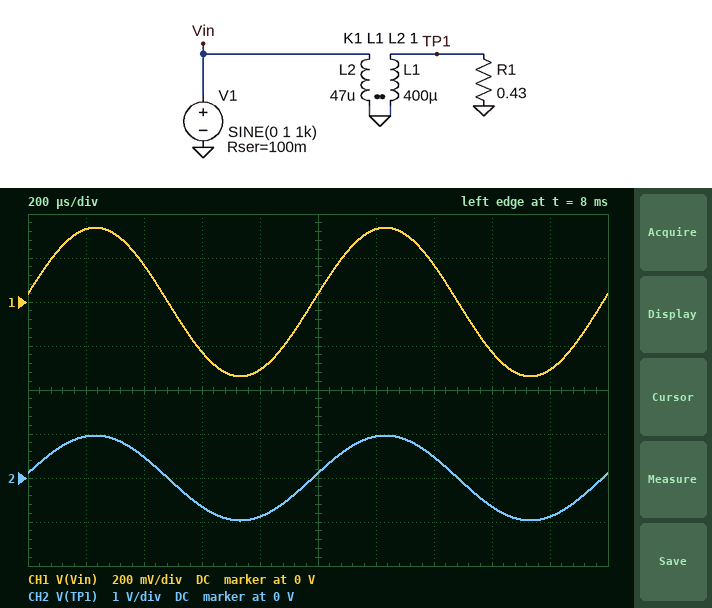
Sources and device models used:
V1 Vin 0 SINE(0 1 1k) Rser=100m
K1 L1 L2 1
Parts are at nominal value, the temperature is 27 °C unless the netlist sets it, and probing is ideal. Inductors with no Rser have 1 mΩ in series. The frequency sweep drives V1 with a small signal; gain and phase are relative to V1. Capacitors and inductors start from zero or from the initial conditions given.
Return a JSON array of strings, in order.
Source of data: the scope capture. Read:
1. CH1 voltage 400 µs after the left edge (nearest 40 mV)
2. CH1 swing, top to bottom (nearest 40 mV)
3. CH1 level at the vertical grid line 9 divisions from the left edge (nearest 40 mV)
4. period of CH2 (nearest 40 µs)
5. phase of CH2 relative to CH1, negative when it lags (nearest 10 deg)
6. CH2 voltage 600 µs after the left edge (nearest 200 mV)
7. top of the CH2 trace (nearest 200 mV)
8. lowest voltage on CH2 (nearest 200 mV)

["160 mV", "680 mV", "-320 mV", "1.00 ms", "0 deg", "-600 mV", "1.0 V", "-1.0 V"]
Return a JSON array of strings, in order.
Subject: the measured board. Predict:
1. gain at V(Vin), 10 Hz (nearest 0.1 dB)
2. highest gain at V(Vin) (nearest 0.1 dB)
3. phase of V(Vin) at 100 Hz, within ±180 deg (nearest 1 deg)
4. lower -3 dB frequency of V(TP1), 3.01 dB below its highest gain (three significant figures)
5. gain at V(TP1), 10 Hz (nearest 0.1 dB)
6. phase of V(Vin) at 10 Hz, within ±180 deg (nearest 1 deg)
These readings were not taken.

["-30.1 dB", "-9.4 dB", "47 deg", "114 Hz", "-21.4 dB", "67 deg"]
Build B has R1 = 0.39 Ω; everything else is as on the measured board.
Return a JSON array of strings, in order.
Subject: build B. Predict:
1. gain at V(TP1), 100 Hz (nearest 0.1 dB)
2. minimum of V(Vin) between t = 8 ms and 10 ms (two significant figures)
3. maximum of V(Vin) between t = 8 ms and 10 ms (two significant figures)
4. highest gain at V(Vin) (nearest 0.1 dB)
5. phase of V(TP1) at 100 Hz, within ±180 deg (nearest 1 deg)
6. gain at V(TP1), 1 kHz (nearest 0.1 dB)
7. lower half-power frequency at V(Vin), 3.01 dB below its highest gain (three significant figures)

["-4.1 dB", "-320 mV", "320 mV", "-9.9 dB", "47 deg", "-0.9 dB", "107 Hz"]
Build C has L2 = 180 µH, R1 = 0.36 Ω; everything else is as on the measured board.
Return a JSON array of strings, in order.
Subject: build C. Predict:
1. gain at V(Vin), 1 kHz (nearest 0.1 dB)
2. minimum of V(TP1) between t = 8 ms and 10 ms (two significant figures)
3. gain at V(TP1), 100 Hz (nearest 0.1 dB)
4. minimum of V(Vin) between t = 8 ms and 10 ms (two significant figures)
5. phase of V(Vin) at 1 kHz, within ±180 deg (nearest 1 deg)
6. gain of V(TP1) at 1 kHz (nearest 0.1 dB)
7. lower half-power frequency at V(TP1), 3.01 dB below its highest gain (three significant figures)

["-4.2 dB", "-920 mV", "-1.9 dB", "-620 mV", "3 deg", "-0.8 dB", "55.1 Hz"]
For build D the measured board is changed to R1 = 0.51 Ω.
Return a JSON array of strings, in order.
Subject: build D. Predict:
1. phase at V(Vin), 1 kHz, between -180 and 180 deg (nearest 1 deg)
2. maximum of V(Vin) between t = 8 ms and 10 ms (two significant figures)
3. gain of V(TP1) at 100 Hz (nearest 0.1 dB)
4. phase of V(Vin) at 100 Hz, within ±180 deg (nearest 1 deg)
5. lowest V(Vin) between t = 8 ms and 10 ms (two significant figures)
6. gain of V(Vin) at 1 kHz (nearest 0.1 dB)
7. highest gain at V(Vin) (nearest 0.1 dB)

["7 deg", "380 mV", "-3.5 dB", "50 deg", "-380 mV", "-8.5 dB", "-8.4 dB"]
